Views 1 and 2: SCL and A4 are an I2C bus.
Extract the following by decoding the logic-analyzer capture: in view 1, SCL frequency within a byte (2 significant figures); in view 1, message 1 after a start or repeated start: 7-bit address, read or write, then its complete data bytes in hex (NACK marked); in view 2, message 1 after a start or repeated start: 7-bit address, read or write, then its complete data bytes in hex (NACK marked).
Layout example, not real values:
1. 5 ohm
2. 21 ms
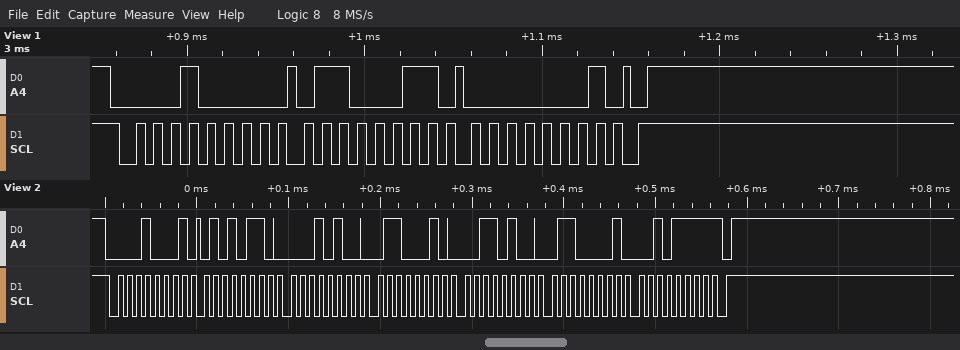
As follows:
1. 100 kHz
2. 0x08 write: 63 01
3. 0x08 read: 56 14 62 34 61 2F NACK
